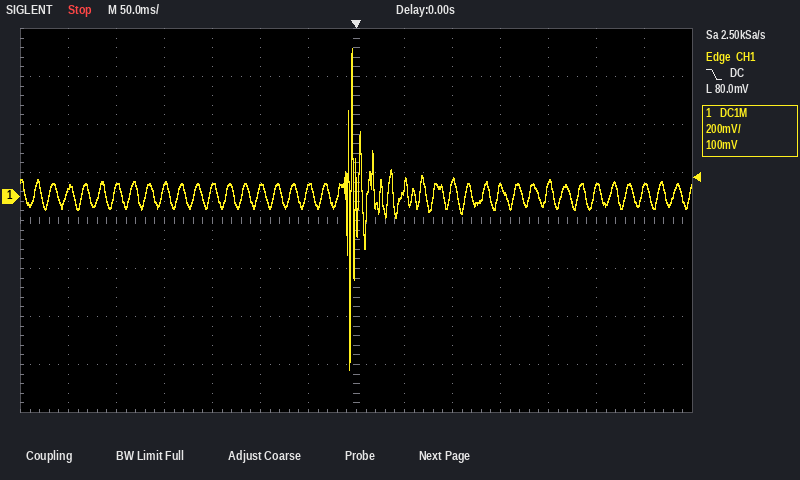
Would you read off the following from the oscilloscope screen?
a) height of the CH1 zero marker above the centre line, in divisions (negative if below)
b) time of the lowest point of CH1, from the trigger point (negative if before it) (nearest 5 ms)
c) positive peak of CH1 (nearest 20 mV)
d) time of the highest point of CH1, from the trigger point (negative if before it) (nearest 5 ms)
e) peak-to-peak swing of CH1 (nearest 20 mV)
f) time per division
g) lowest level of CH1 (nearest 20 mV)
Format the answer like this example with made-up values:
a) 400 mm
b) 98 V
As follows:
a) +0.5 div
b) -5 ms
c) 620 mV
d) -5 ms
e) 1.34 V
f) 50 ms
g) -720 mV
